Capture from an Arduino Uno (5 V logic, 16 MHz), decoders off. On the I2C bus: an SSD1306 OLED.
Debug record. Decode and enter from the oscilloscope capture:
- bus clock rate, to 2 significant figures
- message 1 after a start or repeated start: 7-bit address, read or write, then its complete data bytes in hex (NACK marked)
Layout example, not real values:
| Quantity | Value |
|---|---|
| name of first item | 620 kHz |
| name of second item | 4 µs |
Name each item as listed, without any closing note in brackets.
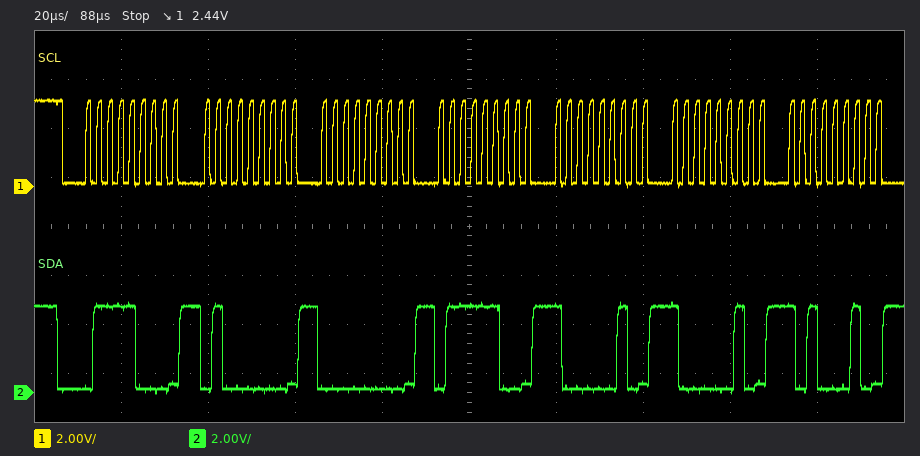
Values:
| Quantity | Value |
|---|---|
| bus clock rate, to 2 significant figures | 400 kHz |
| message 1 after a start or repeated start: 7-bit address, read or write, then its complete data bytes in hex | 0x3C write: 40 00 7C 82 82 A2 |
